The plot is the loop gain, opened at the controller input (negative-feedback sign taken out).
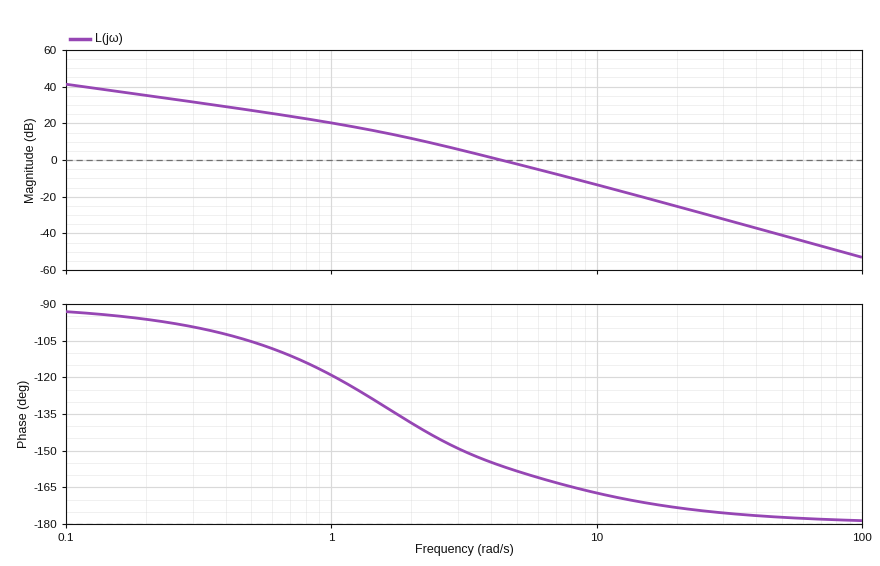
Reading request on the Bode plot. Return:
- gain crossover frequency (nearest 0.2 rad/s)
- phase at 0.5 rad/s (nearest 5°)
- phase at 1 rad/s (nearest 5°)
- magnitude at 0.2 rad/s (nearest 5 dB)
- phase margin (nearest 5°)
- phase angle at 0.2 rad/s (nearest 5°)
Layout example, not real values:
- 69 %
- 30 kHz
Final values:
- 4.4 rad/s
- -105°
- -120°
- 35 dB
- 25°
- -95°
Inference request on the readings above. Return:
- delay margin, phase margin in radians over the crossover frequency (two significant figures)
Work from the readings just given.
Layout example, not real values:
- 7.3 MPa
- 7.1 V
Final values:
- 0.099 s
